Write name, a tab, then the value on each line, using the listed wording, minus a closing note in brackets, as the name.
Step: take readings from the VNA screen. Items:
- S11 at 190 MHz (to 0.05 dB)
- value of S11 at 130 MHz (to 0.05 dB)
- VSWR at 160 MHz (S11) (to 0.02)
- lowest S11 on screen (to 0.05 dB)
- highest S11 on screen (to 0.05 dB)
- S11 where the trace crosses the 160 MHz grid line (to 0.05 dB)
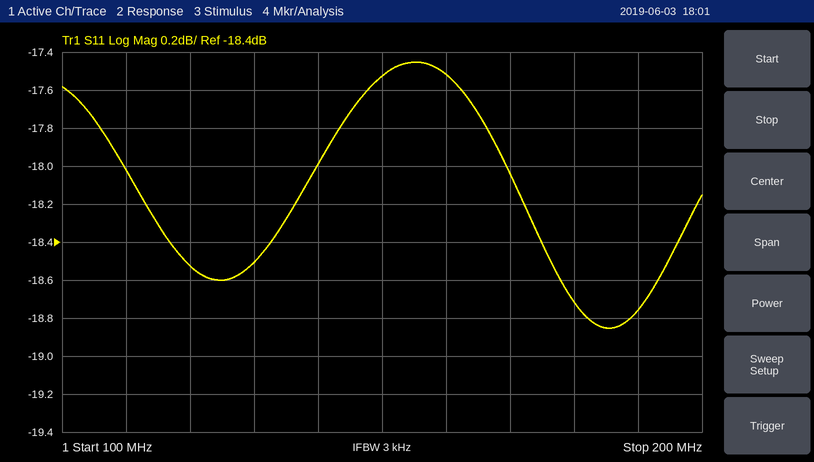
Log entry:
S11 at 190 MHz	-18.75 dB
value of S11 at 130 MHz	-18.50 dB
VSWR at 160 MHz (S11)	1.30
lowest S11 on screen	-18.85 dB
highest S11 on screen	-17.45 dB
S11 where the trace crosses the 160 MHz grid line	-17.50 dB
